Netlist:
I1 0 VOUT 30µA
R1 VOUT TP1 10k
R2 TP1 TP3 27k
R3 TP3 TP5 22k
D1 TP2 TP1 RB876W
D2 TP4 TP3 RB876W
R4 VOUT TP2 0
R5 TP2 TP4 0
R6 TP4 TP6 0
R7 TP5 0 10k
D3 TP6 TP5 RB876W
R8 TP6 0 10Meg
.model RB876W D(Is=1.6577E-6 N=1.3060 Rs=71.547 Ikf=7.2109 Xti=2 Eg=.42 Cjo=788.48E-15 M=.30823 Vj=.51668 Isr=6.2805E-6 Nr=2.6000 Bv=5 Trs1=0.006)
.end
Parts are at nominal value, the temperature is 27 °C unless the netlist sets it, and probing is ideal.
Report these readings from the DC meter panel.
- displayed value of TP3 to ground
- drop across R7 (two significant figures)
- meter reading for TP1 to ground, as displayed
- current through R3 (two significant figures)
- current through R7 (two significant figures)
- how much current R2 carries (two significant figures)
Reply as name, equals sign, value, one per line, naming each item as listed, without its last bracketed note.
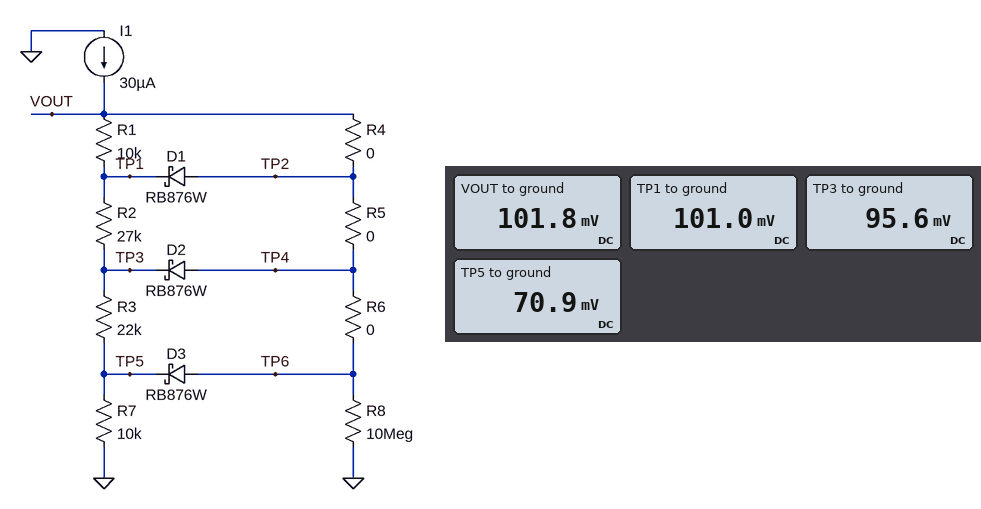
displayed value of TP3 to ground = 95.6 mV
drop across R7 = 71 mV
meter reading for TP1 to ground, as displayed = 101.0 mV
current through R3 = 1.1 µA
current through R7 = 7.1 µA
how much current R2 carries = 200 nA
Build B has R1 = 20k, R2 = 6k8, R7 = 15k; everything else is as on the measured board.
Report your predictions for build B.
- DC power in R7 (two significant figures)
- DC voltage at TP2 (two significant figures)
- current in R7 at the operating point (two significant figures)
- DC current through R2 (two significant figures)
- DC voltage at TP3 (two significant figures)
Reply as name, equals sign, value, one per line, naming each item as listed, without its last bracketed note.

DC power in R7 = 26 µW
DC voltage at TP2 = 720 mV
current in R7 at the operating point = 42 µA
DC current through R2 = 1.2 µA
DC voltage at TP3 = 710 mV
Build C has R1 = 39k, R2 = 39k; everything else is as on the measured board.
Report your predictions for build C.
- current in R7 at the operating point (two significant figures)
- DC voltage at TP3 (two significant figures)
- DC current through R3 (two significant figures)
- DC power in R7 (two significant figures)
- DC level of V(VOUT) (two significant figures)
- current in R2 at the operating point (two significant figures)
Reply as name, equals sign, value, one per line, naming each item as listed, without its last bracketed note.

current in R7 at the operating point = 18 µA
DC voltage at TP3 = 220 mV
DC current through R3 = 2.1 µA
DC power in R7 = 3.1 µW
DC level of V(VOUT) = 230 mV
current in R2 at the operating point = 260 nA
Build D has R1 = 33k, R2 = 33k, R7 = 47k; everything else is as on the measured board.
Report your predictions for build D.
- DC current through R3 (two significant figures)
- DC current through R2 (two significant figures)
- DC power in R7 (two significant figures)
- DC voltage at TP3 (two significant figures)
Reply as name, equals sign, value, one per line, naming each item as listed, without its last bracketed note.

DC current through R3 = 780 nA
DC current through R2 = 120 nA
DC power in R7 = 970 nW
DC voltage at TP3 = 230 mV
